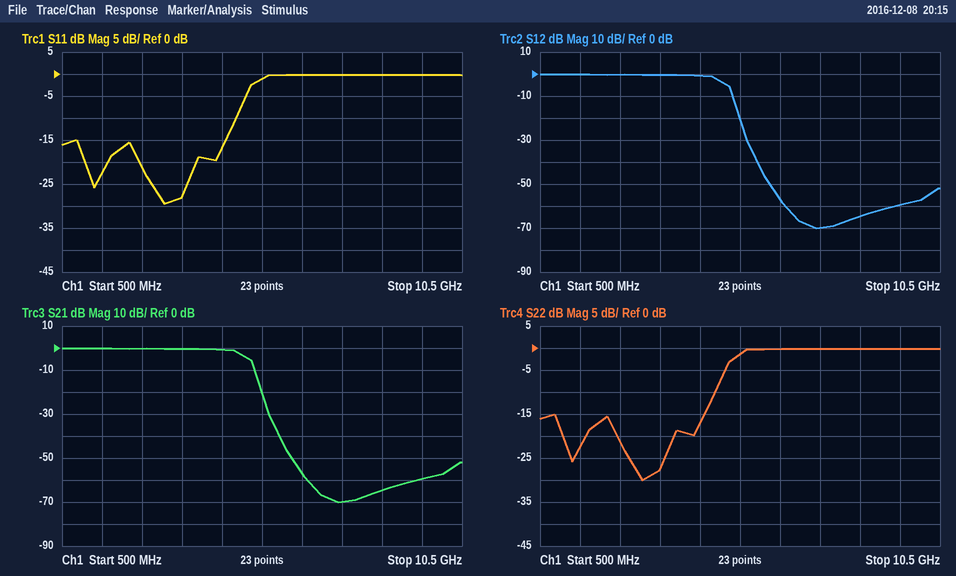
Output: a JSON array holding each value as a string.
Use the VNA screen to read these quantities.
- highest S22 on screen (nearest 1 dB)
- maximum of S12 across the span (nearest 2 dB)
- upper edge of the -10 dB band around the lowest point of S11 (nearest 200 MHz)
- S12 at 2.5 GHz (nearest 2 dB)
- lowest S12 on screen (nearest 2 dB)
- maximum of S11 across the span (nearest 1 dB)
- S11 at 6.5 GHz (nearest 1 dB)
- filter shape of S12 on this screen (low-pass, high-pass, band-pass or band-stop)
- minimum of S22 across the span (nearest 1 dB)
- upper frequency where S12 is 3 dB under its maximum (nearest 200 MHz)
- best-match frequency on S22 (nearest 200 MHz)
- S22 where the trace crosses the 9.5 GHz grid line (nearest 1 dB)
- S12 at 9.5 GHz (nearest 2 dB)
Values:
["0 dB", "0 dB", "4.8 GHz", "0 dB", "-70 dB", "0 dB", "0 dB", "low-pass", "-30 dB", "5.0 GHz", "3.0 GHz", "0 dB", "-60 dB"]
